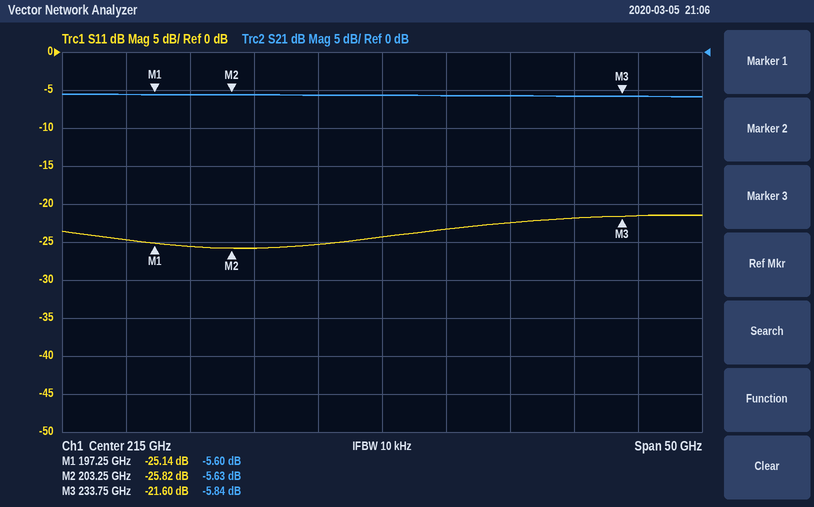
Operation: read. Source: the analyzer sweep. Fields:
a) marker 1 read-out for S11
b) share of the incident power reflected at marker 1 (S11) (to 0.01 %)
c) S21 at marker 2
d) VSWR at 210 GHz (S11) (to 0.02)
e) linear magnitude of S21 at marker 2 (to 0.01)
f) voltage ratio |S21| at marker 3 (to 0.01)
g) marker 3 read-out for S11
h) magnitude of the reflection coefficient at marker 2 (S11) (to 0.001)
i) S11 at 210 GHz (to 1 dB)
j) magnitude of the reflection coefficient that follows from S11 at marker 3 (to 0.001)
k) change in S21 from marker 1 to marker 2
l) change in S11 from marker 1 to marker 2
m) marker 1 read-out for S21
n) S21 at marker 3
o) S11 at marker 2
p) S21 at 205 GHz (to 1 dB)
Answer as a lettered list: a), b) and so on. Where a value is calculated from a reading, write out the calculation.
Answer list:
a) -25.14 dB
b) 10^(-25.14/10) ≈ 0.31 %
c) -5.63 dB
d) |Γ| = 10^(-25/20) = 0.0562; VSWR = (1 + 0.0562)/(1 − 0.0562) ≈ 1.12
e) 10^(-5.63/20) ≈ 0.52
f) 10^(-5.84/20) ≈ 0.51
g) -21.60 dB
h) 10^(-25.82/20) ≈ 0.051
i) -25 dB
j) 10^(-21.6/20) ≈ 0.083
k) -5.63 − (-5.6) = -0.03 dB
l) -25.82 − (-25.14) = -0.68 dB
m) -5.60 dB
n) -5.84 dB
o) -25.82 dB
p) -6 dB
